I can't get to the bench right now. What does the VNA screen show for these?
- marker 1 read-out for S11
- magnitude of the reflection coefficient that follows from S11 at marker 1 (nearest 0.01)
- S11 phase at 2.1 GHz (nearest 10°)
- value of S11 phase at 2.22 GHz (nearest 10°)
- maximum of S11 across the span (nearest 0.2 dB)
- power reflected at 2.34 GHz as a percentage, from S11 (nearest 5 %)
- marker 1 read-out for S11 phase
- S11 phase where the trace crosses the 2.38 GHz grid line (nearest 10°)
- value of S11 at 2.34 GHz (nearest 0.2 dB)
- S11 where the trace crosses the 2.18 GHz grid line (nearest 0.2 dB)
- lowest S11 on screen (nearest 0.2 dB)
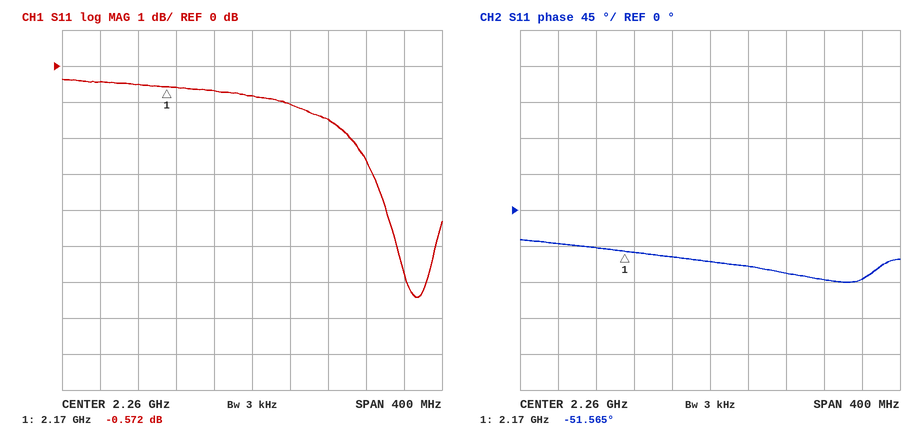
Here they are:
-0.572 dB
0.94
-40°
-60°
-0.4 dB
70 %
-51.565°
-90°
-1.4 dB
-0.6 dB
-6.4 dB
